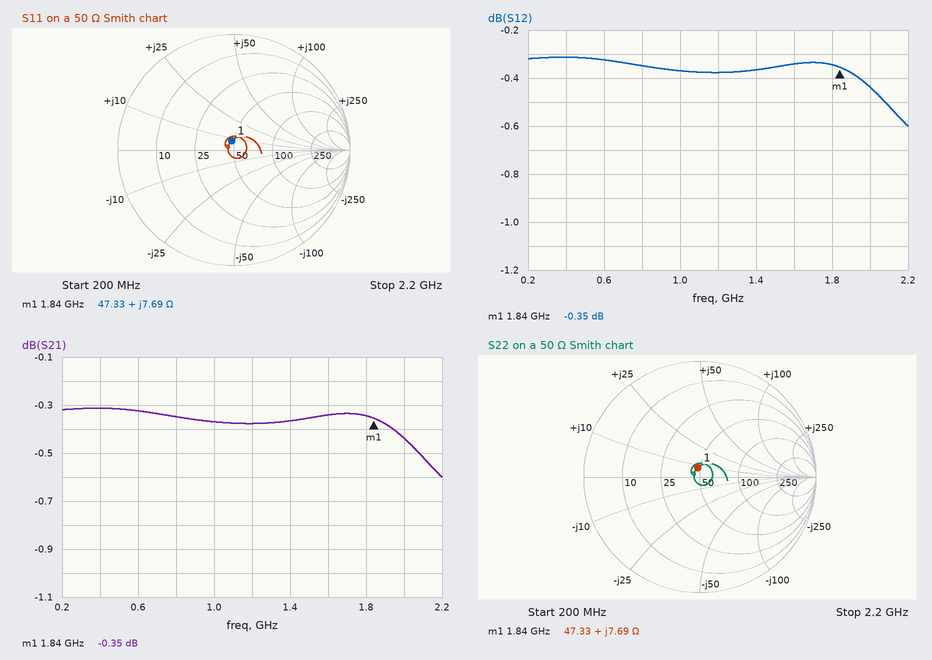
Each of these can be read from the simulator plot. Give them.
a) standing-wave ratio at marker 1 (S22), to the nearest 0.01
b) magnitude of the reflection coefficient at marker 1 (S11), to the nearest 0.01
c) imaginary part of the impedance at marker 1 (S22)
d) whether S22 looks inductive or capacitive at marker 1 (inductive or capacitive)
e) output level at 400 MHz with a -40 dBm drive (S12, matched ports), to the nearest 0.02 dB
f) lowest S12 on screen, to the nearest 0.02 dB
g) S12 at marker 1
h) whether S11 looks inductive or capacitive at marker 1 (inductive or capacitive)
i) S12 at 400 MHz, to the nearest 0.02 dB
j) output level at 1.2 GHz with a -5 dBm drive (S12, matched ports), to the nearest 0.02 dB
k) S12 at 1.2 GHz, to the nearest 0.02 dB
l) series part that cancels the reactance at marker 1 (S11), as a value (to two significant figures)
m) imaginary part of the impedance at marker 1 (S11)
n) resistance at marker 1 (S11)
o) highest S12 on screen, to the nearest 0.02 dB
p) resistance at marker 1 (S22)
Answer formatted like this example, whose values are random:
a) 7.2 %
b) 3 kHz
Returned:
a) 1.18
b) 0.08
c) +7.69 Ω
d) inductive
e) -40.32 dBm
f) -0.60 dB
g) -0.35 dB
h) inductive
i) -0.32 dB
j) -5.38 dBm
k) -0.38 dB
l) 11 pF
m) +7.69 Ω
n) 47.33 Ω
o) -0.32 dB
p) 47.33 Ω
